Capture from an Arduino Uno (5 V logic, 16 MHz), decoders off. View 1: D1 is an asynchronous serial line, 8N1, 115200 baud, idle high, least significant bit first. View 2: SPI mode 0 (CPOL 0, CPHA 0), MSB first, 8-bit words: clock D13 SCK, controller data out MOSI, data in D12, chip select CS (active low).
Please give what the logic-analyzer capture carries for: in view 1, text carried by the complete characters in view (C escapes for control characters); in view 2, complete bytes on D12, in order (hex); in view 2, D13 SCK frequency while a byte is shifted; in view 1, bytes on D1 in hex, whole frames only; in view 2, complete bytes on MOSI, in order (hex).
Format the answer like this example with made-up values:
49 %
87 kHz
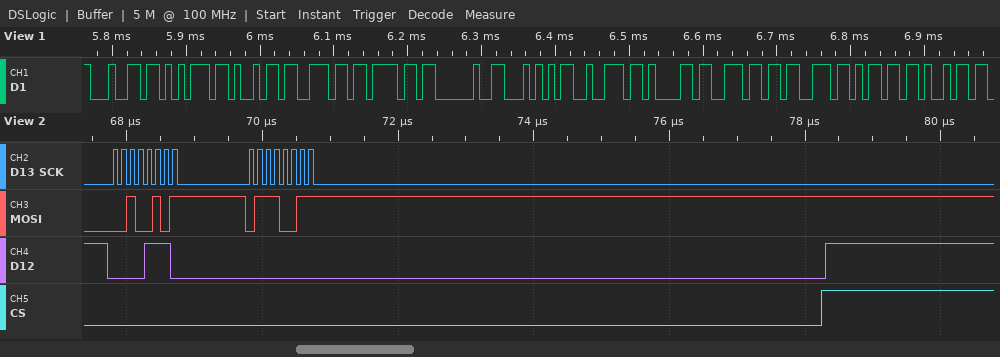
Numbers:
"duino Transmi"
0E 00
8 MHz
64 75 69 6E 6F 20 54 72 61 6E 73 6D 69
25 73
